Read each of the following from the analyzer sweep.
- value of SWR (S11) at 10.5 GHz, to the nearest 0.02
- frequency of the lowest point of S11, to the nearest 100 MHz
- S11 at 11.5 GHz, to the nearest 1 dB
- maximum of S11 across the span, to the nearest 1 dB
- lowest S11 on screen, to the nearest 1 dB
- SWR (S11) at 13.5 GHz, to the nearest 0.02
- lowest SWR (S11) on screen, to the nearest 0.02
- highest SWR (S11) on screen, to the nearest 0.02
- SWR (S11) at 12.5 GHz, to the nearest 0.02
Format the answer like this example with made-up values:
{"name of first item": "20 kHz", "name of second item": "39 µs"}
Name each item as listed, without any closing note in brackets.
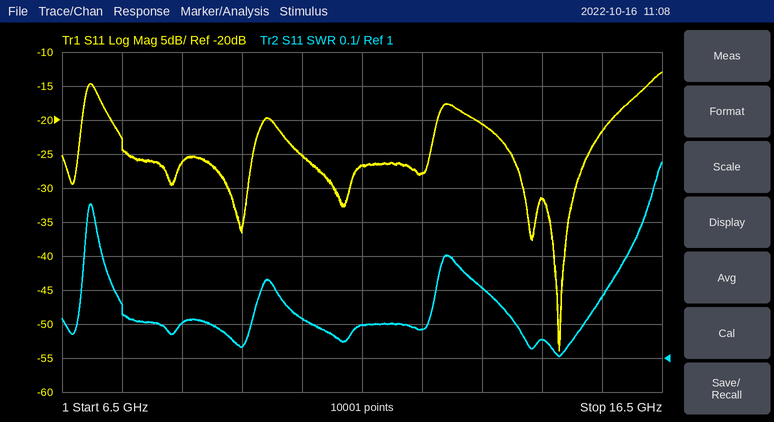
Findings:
{"value of SWR (S11) at 10.5 GHz, to the nearest 0.02": "1.12", "frequency of the lowest point of S11, to the nearest 100 MHz": "14.8 GHz", "S11 at 11.5 GHz, to the nearest 1 dB": "-27 dB", "maximum of S11 across the span, to the nearest 1 dB": "-13 dB", "lowest S11 on screen, to the nearest 1 dB": "-54 dB", "SWR (S11) at 13.5 GHz, to the nearest 0.02": "1.20", "lowest SWR (S11) on screen, to the nearest 0.02": "1.00", "highest SWR (S11) on screen, to the nearest 0.02": "1.58", "SWR (S11) at 12.5 GHz, to the nearest 0.02": "1.08"}
